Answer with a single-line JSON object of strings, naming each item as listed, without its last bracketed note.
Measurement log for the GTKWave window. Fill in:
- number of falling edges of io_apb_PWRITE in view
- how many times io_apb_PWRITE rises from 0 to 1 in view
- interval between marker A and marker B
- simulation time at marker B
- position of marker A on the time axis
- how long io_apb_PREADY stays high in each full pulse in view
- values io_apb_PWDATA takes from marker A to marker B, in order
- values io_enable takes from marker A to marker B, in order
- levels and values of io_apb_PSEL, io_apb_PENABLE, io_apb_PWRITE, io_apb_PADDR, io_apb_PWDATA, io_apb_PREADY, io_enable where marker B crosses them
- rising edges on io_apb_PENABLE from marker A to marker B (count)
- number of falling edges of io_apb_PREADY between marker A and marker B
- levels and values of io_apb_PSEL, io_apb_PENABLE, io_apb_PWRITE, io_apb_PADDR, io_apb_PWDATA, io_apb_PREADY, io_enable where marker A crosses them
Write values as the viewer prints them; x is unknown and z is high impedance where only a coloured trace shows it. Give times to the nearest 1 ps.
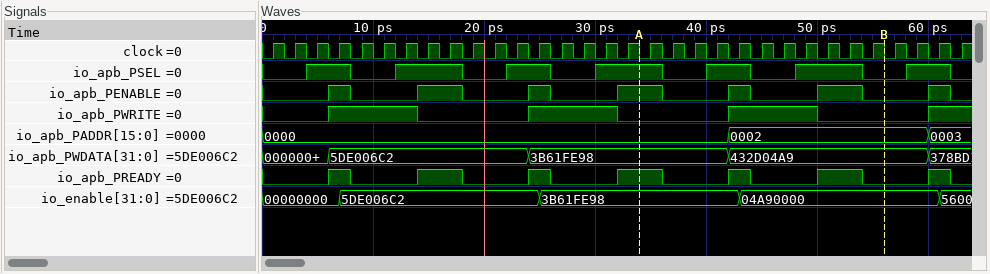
{"number of falling edges of io_apb_PWRITE in view": "3", "how many times io_apb_PWRITE rises from 0 to 1 in view": "4", "interval between marker A and marker B": "22 ps", "simulation time at marker B": "56 ps", "position of marker A on the time axis": "34 ps", "how long io_apb_PREADY stays high in each full pulse in view": "2 ps, 4 ps, 2 ps, 4 ps, 2 ps, 4 ps, 2 ps", "values io_apb_PWDATA takes from marker A to marker B, in order": "3B61FE98, 432D04A9", "values io_enable takes from marker A to marker B, in order": "3B61FE98, 04A90000", "levels and values of io_apb_PSEL, io_apb_PENABLE, io_apb_PWRITE, io_apb_PADDR, io_apb_PWDATA, io_apb_PREADY, io_enable where marker B crosses them": "io_apb_PSEL=0, io_apb_PENABLE=0, io_apb_PWRITE=0, io_apb_PADDR=0002, io_apb_PWDATA=432D04A9, io_apb_PREADY=0, io_enable=04A90000", "rising edges on io_apb_PENABLE from marker A to marker B": "2", "number of falling edges of io_apb_PREADY between marker A and marker B": "3", "levels and values of io_apb_PSEL, io_apb_PENABLE, io_apb_PWRITE, io_apb_PADDR, io_apb_PWDATA, io_apb_PREADY, io_enable where marker A crosses them": "io_apb_PSEL=1, io_apb_PENABLE=1, io_apb_PWRITE=0, io_apb_PADDR=0000, io_apb_PWDATA=3B61FE98, io_apb_PREADY=1, io_enable=3B61FE98"}
